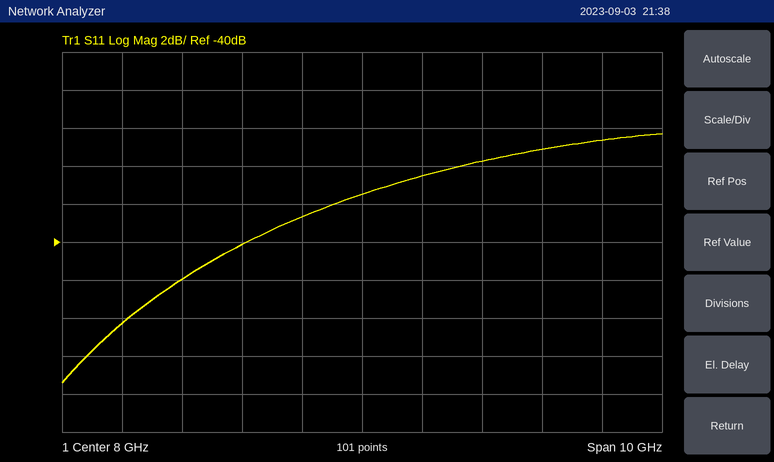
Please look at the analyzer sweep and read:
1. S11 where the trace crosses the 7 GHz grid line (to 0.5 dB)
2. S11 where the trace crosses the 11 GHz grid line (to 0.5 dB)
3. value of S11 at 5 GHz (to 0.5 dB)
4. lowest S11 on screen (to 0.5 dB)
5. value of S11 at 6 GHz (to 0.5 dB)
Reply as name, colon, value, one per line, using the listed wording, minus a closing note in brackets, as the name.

S11 where the trace crosses the 7 GHz grid line: -38.5 dB
S11 where the trace crosses the 11 GHz grid line: -35.0 dB
value of S11 at 5 GHz: -42.0 dB
lowest S11 on screen: -47.5 dB
value of S11 at 6 GHz: -40.0 dB
